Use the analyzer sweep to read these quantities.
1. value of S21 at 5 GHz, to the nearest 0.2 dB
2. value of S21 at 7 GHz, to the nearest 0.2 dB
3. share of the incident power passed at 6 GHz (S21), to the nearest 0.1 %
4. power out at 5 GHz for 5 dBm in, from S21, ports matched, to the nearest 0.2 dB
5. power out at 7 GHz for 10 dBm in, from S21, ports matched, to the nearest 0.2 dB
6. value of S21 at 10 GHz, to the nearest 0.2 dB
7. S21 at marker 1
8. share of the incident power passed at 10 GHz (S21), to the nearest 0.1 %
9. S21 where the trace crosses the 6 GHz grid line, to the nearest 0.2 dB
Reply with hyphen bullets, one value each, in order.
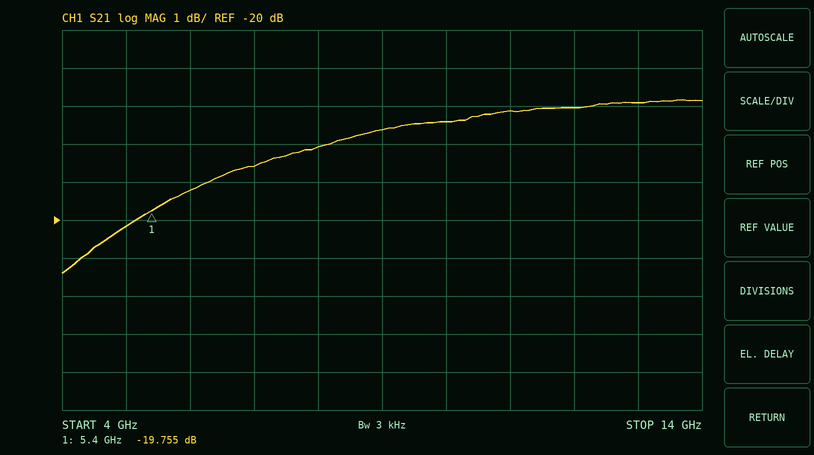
- -20.2 dB
- -18.6 dB
- 1.2 %
- -15.2 dBm
- -8.6 dBm
- -17.4 dB
- -19.755 dB
- 1.8 %
- -19.2 dB
